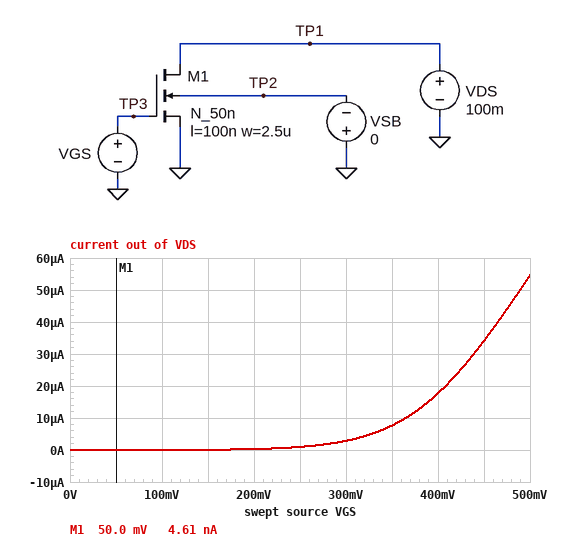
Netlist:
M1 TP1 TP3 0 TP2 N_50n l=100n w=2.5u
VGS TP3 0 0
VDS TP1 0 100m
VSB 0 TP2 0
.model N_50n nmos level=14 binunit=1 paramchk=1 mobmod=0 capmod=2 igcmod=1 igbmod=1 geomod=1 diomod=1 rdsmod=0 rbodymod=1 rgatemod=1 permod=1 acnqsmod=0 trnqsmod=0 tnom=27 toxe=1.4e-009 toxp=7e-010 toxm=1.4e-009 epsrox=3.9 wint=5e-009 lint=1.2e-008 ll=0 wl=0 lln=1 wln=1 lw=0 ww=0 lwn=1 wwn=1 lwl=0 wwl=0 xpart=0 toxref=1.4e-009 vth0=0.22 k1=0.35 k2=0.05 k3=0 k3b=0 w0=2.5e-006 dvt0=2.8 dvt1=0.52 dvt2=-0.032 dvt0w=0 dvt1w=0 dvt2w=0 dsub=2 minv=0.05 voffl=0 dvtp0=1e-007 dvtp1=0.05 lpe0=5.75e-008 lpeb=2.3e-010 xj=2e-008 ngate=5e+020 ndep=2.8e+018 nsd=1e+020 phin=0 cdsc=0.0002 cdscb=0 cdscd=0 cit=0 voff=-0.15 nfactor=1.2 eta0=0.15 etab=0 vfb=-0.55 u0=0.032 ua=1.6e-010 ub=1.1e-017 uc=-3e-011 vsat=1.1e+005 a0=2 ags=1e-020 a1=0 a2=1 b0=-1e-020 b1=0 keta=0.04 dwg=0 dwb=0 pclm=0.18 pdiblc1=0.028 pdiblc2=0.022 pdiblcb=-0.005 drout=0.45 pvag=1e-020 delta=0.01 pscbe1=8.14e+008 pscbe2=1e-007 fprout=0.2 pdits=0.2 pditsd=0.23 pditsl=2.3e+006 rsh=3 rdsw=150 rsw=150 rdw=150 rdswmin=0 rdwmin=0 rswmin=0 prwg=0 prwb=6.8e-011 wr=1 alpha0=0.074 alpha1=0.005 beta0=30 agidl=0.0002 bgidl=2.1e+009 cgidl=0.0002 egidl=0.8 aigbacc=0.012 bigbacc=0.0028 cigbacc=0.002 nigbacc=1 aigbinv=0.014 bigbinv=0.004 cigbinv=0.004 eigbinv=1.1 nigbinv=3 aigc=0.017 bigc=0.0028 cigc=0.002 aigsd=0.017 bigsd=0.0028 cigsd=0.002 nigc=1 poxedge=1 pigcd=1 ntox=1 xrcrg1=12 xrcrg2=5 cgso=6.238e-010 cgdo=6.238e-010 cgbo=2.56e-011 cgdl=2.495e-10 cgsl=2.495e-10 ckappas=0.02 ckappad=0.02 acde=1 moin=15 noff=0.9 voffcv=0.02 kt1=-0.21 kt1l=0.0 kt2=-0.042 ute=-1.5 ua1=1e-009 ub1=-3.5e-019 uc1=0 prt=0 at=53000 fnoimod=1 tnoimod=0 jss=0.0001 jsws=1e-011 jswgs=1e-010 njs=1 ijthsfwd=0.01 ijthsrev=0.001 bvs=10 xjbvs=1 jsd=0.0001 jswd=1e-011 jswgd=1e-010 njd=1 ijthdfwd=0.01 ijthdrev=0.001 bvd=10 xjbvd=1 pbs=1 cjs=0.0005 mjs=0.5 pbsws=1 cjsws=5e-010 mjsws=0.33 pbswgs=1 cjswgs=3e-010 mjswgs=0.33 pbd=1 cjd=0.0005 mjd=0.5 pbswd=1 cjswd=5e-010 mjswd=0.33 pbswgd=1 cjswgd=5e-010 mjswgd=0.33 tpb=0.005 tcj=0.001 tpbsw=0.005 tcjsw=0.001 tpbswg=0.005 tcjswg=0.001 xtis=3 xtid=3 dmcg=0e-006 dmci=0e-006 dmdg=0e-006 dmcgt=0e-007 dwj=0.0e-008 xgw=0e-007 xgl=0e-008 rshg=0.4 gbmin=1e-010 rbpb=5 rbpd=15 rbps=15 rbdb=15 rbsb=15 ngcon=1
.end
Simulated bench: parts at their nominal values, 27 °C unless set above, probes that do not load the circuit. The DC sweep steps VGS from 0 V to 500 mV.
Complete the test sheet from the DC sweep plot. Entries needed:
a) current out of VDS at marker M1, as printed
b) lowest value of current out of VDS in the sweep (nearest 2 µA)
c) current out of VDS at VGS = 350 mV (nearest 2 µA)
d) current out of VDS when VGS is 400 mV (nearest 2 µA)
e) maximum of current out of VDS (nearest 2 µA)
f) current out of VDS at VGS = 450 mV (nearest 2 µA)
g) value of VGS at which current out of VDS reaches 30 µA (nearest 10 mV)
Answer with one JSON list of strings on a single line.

["4.61 nA", "0 A", "8 µA", "18 µA", "54 µA", "34 µA", "440 mV"]
